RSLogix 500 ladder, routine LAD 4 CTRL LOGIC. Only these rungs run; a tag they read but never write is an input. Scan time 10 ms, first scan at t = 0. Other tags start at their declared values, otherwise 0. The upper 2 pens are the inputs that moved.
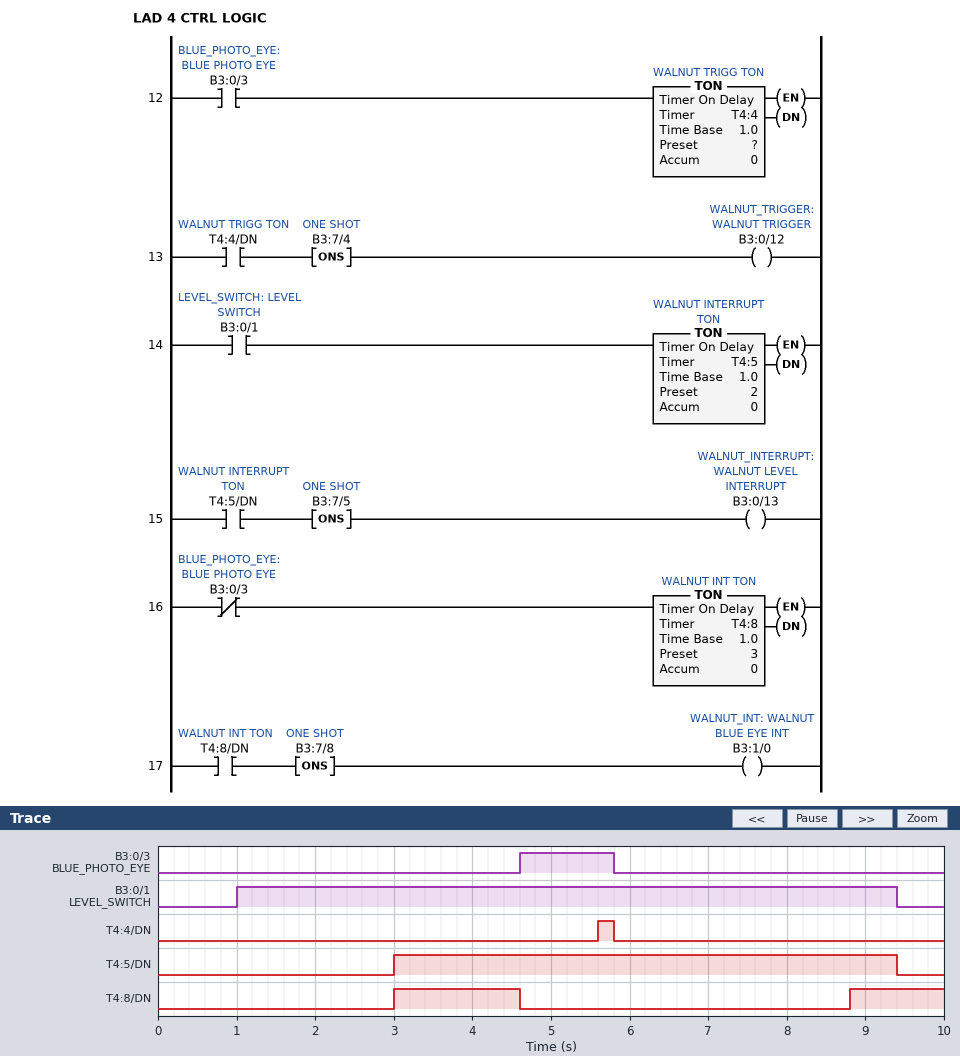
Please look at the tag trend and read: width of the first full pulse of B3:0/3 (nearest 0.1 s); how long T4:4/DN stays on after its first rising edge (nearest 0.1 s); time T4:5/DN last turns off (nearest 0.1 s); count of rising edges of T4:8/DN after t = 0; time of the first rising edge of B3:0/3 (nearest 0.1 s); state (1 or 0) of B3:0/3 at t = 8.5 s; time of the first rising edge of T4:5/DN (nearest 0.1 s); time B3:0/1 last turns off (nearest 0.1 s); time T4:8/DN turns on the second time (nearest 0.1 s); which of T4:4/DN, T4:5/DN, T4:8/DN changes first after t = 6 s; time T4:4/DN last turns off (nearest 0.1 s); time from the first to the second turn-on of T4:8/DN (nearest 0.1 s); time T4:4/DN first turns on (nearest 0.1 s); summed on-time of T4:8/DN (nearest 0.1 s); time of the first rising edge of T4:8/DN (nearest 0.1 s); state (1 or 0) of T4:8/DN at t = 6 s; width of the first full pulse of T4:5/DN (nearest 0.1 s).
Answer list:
1.2 s
0.2 s
9.4 s
2
4.6 s
0
3.0 s
9.4 s
8.8 s
T4:8/DN
5.8 s
5.8 s
5.6 s
2.8 s
3.0 s
0
6.4 s
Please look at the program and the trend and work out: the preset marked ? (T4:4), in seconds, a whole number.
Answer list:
1 s
